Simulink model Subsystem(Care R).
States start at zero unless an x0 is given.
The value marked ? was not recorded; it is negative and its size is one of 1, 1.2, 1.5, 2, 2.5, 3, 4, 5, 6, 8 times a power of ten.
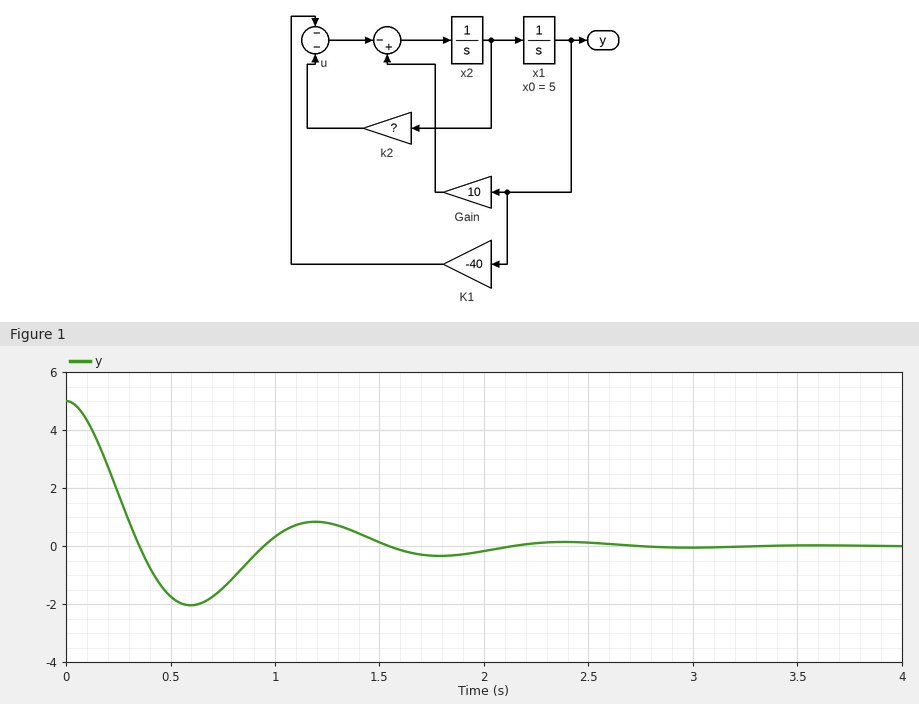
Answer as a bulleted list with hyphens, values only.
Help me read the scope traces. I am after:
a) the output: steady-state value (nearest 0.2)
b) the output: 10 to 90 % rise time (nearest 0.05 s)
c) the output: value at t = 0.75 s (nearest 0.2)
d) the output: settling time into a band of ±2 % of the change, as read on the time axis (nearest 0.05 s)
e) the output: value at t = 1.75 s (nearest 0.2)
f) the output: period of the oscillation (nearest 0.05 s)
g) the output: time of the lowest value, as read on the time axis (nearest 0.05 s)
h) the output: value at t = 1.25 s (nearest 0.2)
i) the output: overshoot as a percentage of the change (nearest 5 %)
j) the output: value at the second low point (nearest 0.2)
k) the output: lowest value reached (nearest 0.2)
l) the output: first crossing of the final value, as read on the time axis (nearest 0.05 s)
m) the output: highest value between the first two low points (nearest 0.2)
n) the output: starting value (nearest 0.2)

- 0.0
- 0.25 s
- -1.4
- 2.55 s
- -0.4
- 1.20 s
- 0.60 s
- 0.8
- 40 %
- -0.4
- -2.0
- 0.35 s
- 0.8
- 5.0
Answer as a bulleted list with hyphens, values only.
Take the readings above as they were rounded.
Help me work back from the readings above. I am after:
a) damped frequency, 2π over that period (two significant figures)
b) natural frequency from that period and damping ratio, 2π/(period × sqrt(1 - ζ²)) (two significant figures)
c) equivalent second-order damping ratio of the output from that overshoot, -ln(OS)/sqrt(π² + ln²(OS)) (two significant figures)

- 5.2 rad/s
- 5.5 rad/s
- 0.28
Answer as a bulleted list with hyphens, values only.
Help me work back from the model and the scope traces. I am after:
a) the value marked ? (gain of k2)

- -3
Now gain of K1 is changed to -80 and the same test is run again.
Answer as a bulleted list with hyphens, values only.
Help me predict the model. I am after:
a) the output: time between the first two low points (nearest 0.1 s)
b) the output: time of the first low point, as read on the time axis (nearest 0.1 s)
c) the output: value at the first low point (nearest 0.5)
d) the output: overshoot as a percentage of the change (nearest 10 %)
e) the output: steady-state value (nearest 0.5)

- 0.8 s
- 0.4 s
- -3.0
- 60 %
- 0.0
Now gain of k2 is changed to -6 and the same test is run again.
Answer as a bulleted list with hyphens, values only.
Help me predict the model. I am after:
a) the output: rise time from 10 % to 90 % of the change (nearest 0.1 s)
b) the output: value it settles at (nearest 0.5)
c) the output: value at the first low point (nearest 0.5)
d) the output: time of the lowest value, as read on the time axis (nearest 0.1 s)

- 0.3 s
- 0.0
- -0.5
- 0.7 s
